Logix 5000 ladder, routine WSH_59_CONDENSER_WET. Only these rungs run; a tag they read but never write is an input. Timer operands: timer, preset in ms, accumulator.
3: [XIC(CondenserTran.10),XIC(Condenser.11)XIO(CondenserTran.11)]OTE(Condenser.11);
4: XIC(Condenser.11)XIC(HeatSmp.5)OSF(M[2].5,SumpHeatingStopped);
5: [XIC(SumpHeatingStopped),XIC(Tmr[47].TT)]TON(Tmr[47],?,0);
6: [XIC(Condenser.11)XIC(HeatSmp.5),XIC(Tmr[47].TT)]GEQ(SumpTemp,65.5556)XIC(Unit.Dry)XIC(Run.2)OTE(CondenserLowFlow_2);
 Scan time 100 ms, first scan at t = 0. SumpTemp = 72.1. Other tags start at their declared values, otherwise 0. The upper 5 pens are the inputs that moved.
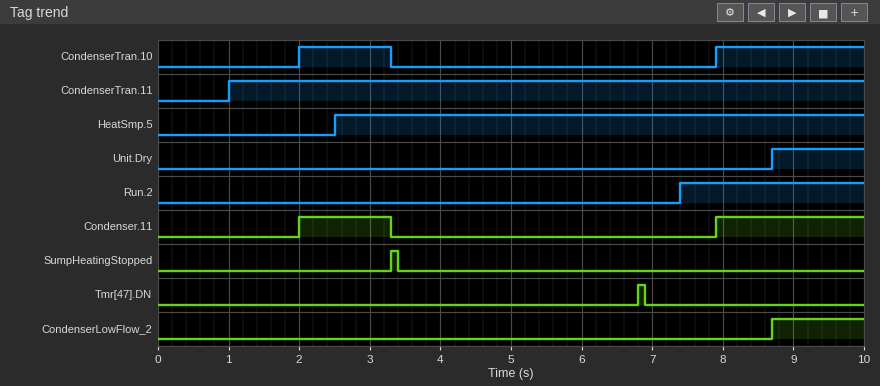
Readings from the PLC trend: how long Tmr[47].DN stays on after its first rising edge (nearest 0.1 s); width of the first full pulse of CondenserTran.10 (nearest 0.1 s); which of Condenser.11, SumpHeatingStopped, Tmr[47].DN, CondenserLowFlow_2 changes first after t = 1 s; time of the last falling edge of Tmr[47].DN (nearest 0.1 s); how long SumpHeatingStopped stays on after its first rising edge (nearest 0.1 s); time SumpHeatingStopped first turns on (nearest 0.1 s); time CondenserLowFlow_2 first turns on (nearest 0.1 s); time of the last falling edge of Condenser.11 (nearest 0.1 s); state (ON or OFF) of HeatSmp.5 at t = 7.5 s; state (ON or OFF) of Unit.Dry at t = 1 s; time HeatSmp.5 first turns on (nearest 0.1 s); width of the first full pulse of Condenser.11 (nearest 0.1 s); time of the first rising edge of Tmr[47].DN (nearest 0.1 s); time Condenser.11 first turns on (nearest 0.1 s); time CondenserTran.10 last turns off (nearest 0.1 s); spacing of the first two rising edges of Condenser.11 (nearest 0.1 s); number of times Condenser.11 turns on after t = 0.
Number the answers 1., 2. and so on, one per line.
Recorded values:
1. 0.1 s
2. 1.3 s
3. Condenser.11
4. 6.9 s
5. 0.1 s
6. 3.3 s
7. 8.7 s
8. 3.3 s
9. ON
10. OFF
11. 2.5 s
12. 1.3 s
13. 6.8 s
14. 2.0 s
15. 3.3 s
16. 5.9 s
17. 2
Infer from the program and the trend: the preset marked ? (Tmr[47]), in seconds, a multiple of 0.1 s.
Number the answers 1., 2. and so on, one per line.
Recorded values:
1. 3.5 s
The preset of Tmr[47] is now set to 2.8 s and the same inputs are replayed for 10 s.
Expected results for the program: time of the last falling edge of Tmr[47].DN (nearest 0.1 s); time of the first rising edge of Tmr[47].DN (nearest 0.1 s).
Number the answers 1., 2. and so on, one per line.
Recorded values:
1. 6.2 s
2. 6.1 s
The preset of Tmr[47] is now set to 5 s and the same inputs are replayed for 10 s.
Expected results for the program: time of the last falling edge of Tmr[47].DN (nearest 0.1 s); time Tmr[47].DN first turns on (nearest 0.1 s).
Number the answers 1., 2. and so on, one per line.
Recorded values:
1. 8.4 s
2. 8.3 s
